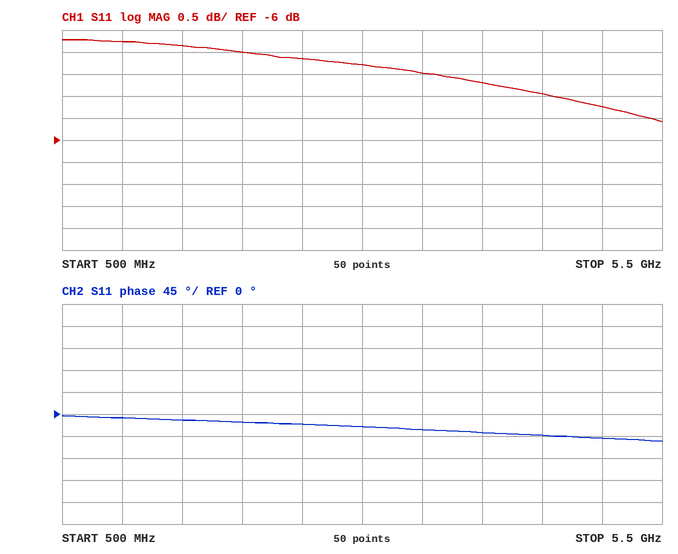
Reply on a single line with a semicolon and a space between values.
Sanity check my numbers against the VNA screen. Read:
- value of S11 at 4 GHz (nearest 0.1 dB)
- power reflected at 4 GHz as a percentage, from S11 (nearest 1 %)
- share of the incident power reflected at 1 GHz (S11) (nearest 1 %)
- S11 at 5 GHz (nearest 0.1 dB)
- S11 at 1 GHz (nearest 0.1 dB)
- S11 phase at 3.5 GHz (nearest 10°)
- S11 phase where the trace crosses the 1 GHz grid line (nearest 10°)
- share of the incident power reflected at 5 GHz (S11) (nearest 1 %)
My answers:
-4.7 dB; 34 %; 42 %; -5.2 dB; -3.8 dB; -30°; -10°; 30 %
